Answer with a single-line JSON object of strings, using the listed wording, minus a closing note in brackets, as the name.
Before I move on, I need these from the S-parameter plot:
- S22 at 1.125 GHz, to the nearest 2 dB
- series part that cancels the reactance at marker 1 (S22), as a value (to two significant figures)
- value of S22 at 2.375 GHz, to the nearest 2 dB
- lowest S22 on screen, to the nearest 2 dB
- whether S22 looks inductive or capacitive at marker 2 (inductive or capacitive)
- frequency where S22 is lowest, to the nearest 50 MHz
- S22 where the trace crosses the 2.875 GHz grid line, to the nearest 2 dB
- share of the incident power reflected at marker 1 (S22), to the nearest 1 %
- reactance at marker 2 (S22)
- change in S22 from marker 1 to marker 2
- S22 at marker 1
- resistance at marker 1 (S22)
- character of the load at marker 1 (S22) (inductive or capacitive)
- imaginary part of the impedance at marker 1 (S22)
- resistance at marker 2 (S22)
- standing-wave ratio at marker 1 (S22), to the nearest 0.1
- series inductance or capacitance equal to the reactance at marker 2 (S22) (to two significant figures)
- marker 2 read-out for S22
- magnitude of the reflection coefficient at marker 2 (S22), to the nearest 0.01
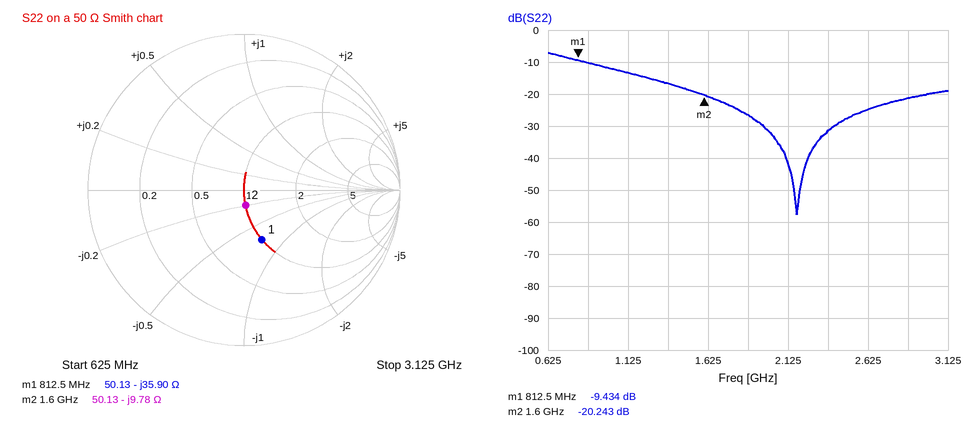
{"S22 at 1.125 GHz, to the nearest 2 dB": "-14 dB", "series part that cancels the reactance at marker 1 (S22), as a value": "7.0 nH", "value of S22 at 2.375 GHz, to the nearest 2 dB": "-32 dB", "lowest S22 on screen, to the nearest 2 dB": "-58 dB", "whether S22 looks inductive or capacitive at marker 2": "capacitive", "frequency where S22 is lowest, to the nearest 50 MHz": "2.20 GHz", "S22 where the trace crosses the 2.875 GHz grid line, to the nearest 2 dB": "-22 dB", "share of the incident power reflected at marker 1 (S22), to the nearest 1 %": "11 %", "reactance at marker 2": "-9.78 Ω", "change in S22 from marker 1 to marker 2": "-10.809 dB", "S22 at marker 1": "-9.434 dB", "resistance at marker 1": "50.13 Ω", "character of the load at marker 1 (S22)": "capacitive", "imaginary part of the impedance at marker 1": "-35.90 Ω", "resistance at marker 2": "50.13 Ω", "standing-wave ratio at marker 1 (S22), to the nearest 0.1": "2.0", "series inductance or capacitance equal to the reactance at marker 2 (S22)": "10 pF", "marker 2 read-out for S22": "-20.243 dB", "magnitude of the reflection coefficient at marker 2 (S22), to the nearest 0.01": "0.10"}
